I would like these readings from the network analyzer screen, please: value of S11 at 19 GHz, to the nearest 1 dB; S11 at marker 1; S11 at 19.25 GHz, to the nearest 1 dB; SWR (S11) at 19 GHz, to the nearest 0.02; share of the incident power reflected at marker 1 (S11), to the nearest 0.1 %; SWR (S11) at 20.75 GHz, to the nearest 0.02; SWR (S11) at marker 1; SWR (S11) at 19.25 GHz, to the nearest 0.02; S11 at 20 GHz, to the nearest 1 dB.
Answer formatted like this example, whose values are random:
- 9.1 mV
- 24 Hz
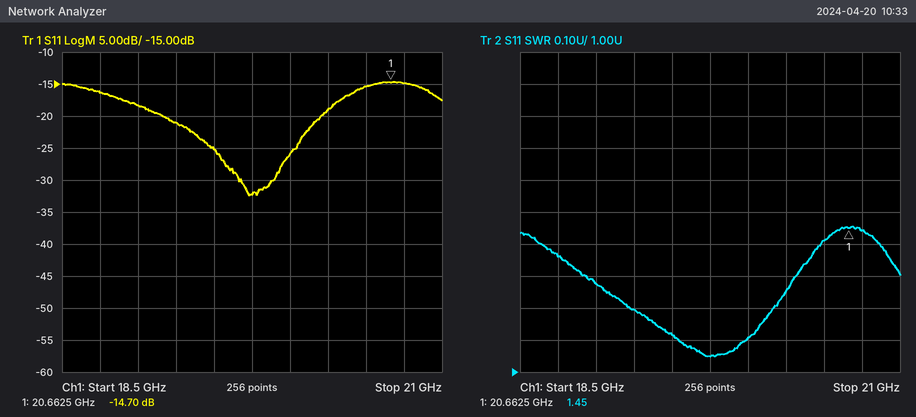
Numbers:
- -18 dB
- -14.70 dB
- -21 dB
- 1.28
- 3.4 %
- 1.44
- 1.45
- 1.20
- -26 dB
